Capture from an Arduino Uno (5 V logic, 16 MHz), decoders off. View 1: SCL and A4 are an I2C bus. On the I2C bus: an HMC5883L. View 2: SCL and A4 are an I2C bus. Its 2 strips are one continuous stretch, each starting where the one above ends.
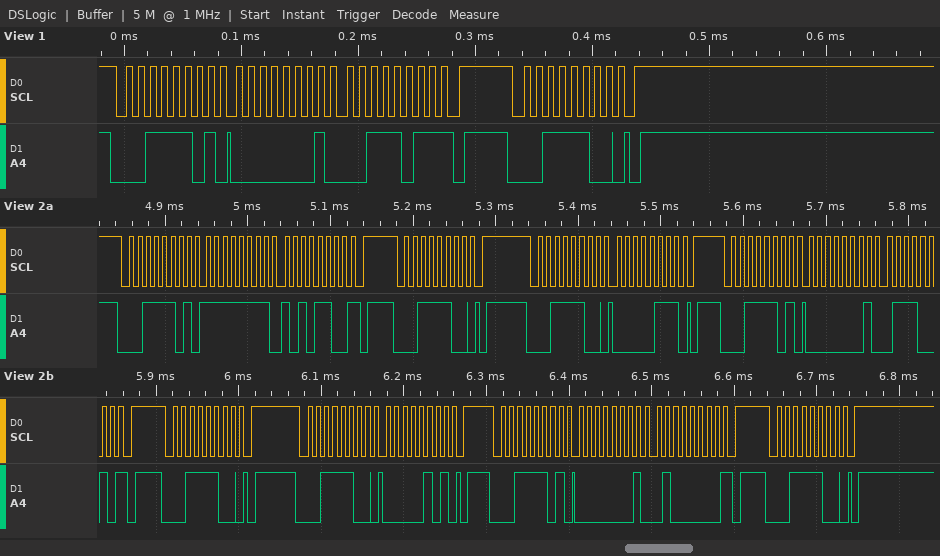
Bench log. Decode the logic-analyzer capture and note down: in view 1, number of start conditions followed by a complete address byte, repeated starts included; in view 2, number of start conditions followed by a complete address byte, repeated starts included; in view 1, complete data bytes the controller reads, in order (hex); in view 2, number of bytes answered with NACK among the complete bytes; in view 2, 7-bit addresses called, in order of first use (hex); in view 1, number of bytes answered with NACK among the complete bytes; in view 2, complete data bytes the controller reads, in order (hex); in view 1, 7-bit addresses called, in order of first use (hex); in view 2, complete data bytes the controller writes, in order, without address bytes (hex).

2
8
01 3B
3
0x1E
1
FF AC 01 72 01 40
0x1E
07 05
